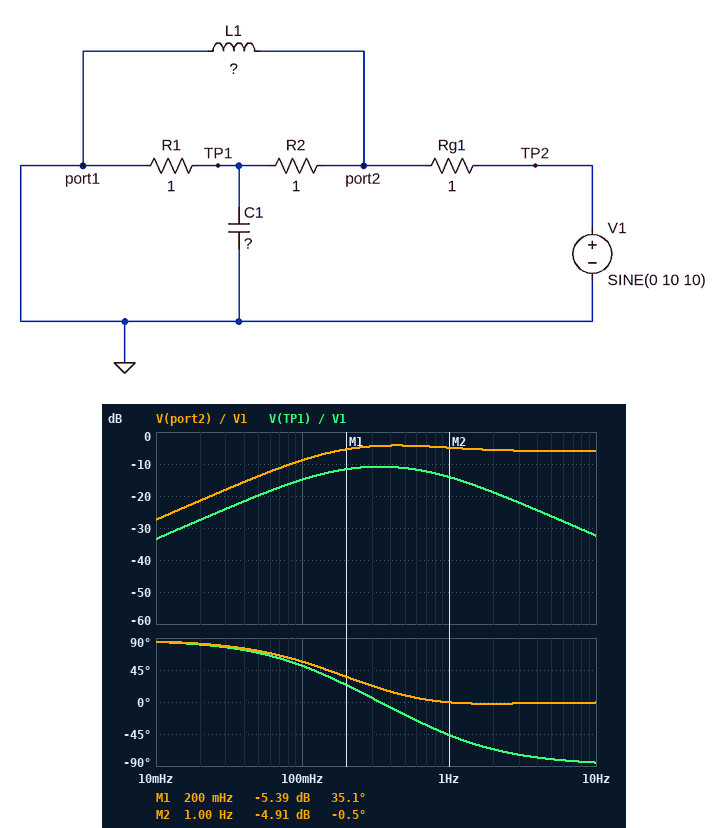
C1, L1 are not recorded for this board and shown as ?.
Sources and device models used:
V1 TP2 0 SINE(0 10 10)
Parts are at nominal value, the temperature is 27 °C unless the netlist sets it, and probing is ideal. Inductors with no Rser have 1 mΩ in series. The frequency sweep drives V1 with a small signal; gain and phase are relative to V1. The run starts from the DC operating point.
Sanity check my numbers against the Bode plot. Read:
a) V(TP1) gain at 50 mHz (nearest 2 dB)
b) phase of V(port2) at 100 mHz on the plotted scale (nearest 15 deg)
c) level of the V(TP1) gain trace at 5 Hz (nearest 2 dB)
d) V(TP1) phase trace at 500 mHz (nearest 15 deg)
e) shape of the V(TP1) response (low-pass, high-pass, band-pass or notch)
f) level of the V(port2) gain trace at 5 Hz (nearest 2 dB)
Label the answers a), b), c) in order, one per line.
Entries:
a) -20 dB
b) 60 deg
c) -26 dB
d) -15 deg
e) band-pass
f) -6 dB
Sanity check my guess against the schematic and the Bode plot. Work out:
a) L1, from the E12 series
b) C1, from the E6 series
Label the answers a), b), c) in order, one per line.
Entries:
a) 680 mH
b) 330 mF
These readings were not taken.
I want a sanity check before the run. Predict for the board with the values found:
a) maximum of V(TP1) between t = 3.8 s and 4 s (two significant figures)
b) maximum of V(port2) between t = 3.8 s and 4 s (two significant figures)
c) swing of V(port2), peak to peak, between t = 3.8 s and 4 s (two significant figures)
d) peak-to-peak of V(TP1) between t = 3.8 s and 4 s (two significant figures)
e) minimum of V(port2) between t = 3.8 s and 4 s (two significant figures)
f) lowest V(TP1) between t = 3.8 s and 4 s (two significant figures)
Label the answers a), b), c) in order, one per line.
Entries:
a) 240 mV
b) 5.0 V
c) 10 V
d) 480 mV
e) -5.0 V
f) -240 mV
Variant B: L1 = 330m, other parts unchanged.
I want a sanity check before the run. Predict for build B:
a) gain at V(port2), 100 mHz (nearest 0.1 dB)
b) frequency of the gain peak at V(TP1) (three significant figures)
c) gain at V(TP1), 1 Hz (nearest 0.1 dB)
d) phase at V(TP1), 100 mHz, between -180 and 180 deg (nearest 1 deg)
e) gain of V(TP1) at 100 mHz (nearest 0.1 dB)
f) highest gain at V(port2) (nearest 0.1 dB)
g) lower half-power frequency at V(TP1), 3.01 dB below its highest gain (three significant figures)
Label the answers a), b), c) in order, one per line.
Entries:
a) -14.0 dB
b) 483 mHz
c) -14.2 dB
d) 66 deg
e) -20.1 dB
f) -4.8 dB
g) 200 mHz
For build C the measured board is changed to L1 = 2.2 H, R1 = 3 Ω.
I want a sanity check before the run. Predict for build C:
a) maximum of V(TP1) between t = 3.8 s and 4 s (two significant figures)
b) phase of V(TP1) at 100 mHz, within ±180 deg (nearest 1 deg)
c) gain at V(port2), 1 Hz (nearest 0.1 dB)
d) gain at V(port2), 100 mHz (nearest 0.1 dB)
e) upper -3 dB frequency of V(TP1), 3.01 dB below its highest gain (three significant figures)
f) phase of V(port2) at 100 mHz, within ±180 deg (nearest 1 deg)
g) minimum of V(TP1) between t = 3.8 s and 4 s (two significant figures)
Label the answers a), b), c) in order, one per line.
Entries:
a) 230 mV
b) 17 deg
c) -5.1 dB
d) -3.0 dB
e) 486 mHz
f) 26 deg
g) -250 mV
